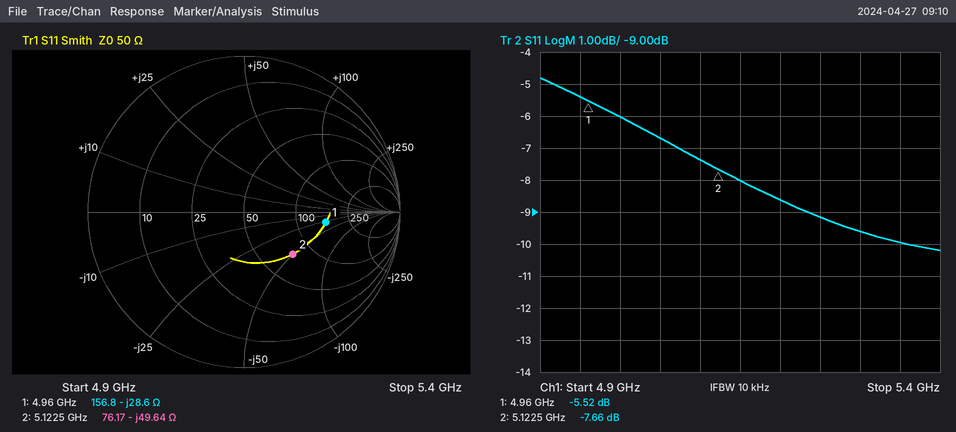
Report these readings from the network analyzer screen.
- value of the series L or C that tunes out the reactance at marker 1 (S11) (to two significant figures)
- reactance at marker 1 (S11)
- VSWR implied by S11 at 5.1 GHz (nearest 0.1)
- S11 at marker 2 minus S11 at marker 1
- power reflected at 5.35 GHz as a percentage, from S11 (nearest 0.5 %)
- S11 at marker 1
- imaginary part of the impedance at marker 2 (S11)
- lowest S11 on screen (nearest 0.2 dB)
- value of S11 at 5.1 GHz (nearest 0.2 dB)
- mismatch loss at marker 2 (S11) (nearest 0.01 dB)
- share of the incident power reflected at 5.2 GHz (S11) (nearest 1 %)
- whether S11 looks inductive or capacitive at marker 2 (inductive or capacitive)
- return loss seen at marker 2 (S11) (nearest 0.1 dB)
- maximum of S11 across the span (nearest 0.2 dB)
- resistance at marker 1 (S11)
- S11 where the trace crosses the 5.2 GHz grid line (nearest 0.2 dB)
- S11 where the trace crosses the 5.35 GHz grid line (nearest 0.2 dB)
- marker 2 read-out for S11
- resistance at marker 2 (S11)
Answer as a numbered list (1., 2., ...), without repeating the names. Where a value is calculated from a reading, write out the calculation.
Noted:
1. L = 28.6 Ω/(2π × 4.96 GHz) ≈ 918 pH, so 920 pH to two significant figures
2. -28.6 Ω
3. |Γ| = 10^(-7.4/20) = 0.4266; VSWR = (1 + 0.4266)/(1 − 0.4266) ≈ 2.5
4. -7.66 − (-5.52) = -2.14 dB
5. 10^(-10/10) ≈ 10.0 %
6. -5.52 dB
7. -49.64 Ω
8. -10.2 dB
9. -7.4 dB
10. −10 log10(1 − 10^(-7.66/10)) ≈ 0.82 dB
11. 10^(-8.6/10) ≈ 14 %
12. capacitive
13. 7.7 dB
14. -4.8 dB
15. 156.8 Ω
16. -8.6 dB
17. -10.0 dB
18. -7.66 dB
19. 76.17 Ω
